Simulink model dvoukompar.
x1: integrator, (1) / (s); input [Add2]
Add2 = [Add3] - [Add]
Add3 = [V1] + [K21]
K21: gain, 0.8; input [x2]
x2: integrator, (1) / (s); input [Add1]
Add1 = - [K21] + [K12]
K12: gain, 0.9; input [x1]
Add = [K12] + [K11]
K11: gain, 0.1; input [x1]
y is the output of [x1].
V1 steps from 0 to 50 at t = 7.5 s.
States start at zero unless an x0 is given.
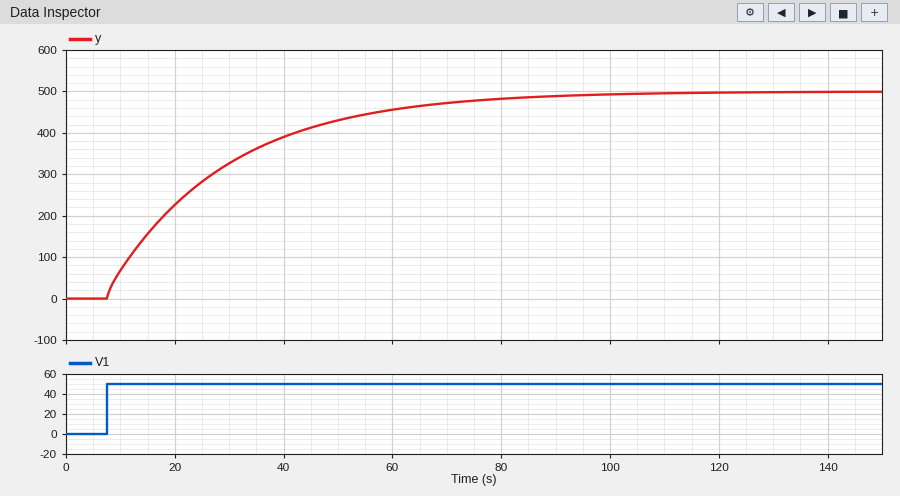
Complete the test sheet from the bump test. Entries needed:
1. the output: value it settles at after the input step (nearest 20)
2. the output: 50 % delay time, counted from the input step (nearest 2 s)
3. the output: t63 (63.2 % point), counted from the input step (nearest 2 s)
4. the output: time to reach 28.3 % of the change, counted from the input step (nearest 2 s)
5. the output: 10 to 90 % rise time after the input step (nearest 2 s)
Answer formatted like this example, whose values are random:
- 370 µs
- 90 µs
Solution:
- 500
- 14 s
- 22 s
- 6 s
- 48 s
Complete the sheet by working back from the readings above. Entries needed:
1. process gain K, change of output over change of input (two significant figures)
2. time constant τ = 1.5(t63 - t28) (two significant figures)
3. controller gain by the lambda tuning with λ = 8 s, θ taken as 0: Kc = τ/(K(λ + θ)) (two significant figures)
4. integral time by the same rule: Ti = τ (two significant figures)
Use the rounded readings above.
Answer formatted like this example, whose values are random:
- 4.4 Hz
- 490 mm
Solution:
- 10
- 24 s
- 0.30
- 24 s
